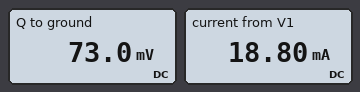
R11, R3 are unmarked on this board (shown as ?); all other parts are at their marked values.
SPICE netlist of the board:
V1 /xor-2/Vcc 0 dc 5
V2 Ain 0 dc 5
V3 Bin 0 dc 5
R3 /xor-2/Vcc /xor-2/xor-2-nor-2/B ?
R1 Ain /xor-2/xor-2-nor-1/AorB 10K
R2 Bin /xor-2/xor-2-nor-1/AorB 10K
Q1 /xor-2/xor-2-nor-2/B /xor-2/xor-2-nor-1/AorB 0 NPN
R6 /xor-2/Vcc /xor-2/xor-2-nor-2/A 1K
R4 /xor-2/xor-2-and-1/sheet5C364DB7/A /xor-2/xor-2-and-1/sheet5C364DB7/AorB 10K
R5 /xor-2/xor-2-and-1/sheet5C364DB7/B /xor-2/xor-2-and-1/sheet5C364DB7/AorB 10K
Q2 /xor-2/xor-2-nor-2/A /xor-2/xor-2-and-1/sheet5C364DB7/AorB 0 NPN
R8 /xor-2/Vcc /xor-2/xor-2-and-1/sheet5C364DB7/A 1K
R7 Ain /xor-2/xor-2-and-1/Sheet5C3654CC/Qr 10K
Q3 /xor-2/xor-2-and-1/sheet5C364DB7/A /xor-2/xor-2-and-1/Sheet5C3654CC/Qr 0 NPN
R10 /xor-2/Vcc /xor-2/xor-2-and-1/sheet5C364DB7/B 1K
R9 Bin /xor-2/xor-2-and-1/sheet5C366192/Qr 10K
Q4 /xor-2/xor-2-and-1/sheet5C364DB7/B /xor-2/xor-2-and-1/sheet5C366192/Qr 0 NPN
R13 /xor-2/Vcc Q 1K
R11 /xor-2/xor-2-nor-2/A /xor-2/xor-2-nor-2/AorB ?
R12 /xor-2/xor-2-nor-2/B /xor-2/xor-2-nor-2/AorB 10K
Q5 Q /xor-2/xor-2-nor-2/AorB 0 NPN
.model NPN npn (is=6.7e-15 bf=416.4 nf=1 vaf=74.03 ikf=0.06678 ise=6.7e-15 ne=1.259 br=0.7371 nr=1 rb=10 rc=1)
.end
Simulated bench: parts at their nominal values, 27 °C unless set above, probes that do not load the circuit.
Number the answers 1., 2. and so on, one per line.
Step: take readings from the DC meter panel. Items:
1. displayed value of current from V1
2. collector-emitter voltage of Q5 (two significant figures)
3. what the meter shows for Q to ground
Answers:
1. 18.80 mA
2. 73 mV
3. 73.0 mV
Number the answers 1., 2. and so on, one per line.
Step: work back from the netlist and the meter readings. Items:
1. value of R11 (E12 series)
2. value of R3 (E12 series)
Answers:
1. 4.7 kΩ
2. 1.5 kΩ
